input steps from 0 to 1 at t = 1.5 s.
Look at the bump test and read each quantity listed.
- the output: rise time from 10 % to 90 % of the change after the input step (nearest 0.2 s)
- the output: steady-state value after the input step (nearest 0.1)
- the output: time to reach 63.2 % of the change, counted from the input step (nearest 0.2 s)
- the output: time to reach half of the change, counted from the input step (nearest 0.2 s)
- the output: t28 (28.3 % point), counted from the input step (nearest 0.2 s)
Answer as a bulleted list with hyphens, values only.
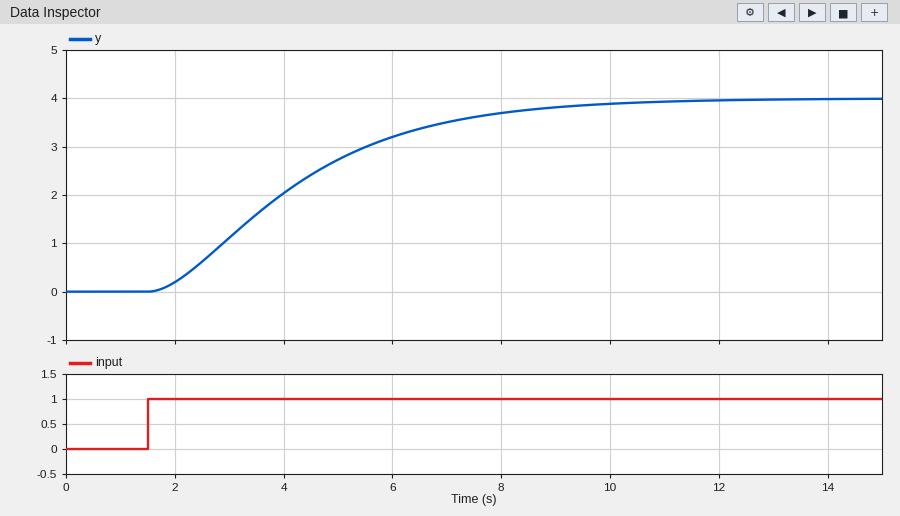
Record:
- 5.2 s
- 4.0
- 3.2 s
- 2.4 s
- 1.6 s
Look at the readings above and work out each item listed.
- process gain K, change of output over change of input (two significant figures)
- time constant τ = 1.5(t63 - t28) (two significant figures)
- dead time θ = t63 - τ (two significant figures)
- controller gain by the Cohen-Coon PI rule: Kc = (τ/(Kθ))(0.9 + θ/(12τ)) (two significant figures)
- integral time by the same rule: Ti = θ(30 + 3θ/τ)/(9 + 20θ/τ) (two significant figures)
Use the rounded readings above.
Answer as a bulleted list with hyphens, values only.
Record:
- 4.0
- 2.4 s
- 0.80 s
- 0.70
- 1.6 s
